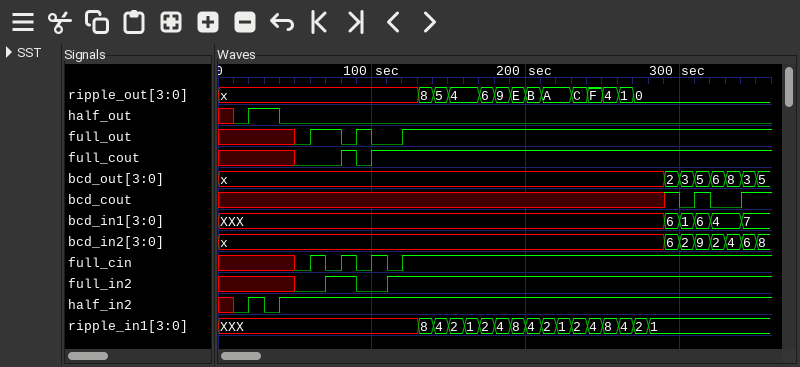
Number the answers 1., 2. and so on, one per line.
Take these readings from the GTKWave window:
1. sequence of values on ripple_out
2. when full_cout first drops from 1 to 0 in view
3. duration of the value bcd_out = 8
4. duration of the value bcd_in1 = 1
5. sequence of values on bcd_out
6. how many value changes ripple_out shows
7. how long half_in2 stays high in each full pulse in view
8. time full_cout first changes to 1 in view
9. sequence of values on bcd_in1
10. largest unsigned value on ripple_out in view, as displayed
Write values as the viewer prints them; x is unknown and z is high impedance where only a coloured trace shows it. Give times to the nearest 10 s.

1. x, 8, 5, 4, 6, 9, E, B, A, C, F, 4, 1, 0
2. 90 s
3. 10 s
4. 10 s
5. x, 2, 3, 5, 6, 8, 3, 5
6. 13
7. 10 s
8. 80 s
9. XXX, 6, 1, 6, 4, 7
10. F
